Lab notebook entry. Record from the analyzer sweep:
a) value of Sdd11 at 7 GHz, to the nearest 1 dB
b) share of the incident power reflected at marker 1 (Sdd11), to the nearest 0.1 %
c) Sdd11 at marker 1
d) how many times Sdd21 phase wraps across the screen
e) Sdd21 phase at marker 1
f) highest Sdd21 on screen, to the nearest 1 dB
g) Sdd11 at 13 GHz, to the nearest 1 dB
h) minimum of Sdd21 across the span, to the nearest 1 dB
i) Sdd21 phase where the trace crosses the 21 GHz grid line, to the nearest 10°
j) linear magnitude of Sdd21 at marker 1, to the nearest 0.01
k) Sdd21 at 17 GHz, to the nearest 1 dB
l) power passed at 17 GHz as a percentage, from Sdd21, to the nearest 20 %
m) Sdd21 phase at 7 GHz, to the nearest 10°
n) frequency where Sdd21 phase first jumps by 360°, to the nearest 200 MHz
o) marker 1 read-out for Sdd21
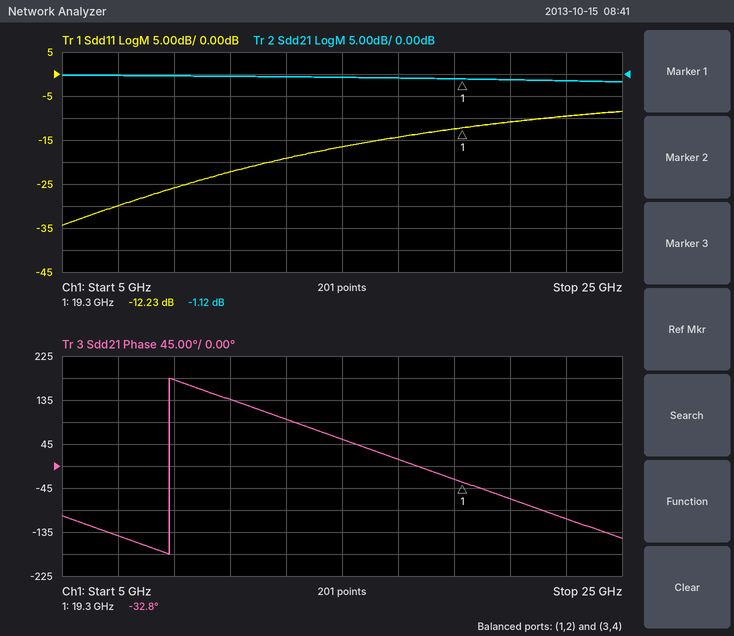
-30 dB
6.0 %
-12.23 dB
1
-32.8°
0 dB
-19 dB
-2 dB
-70°
0.88
-1 dB
80 %
-140°
8.8 GHz
-1.12 dB
